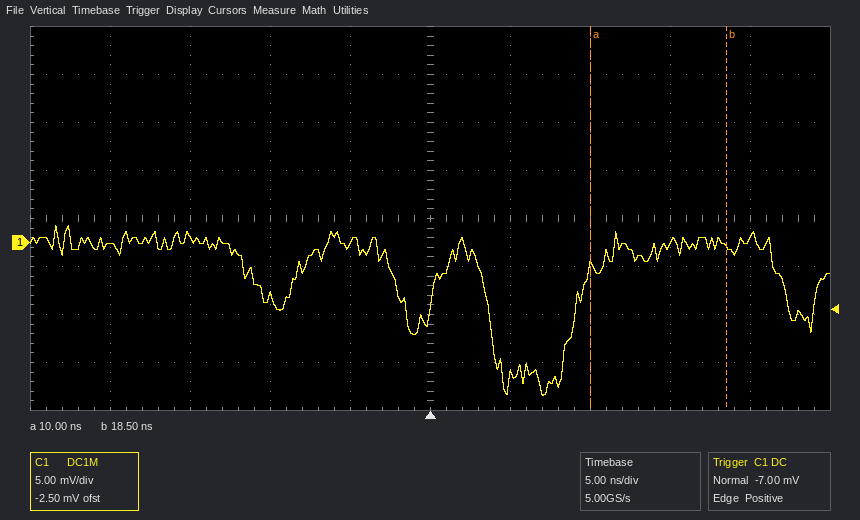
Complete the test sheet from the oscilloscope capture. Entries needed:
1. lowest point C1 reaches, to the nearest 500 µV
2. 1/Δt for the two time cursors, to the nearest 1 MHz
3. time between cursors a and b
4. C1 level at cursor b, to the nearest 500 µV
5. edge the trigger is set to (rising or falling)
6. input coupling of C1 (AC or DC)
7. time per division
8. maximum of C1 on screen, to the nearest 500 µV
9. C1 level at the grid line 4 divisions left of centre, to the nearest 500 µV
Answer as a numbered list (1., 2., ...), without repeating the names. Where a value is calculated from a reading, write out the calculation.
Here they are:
1. -16.0 mV
2. 1 / 8.5 ns ≈ 118 MHz
3. 18.5 ns − (10 ns) = 8.5 ns
4. -500 µV
5. rising
6. DC
7. 5 ns
8. 2.0 mV
9. 0.0 mV
